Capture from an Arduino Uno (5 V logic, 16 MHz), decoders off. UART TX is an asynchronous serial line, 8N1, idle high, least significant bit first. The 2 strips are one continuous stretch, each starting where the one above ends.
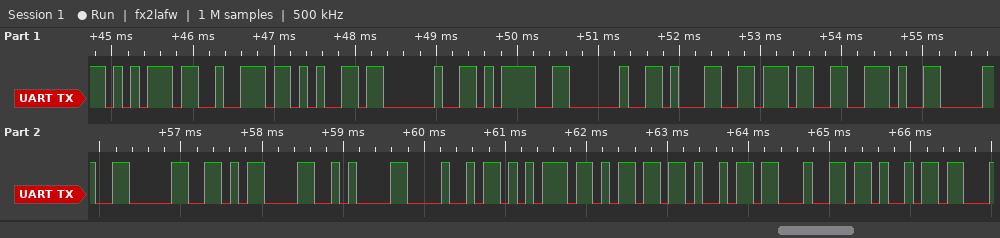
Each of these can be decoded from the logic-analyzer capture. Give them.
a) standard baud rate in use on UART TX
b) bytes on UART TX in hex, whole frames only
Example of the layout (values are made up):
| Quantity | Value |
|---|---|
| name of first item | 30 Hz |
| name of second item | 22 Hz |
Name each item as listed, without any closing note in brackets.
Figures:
| Quantity | Value |
|---|---|
| standard baud rate in use on UART TX | 9600 baud |
| bytes on UART TX in hex, whole frames only | 75 72 65 20 3D 20 31 37 2E 30 30 0D 0A 48 75 6D 69 64 69 |
